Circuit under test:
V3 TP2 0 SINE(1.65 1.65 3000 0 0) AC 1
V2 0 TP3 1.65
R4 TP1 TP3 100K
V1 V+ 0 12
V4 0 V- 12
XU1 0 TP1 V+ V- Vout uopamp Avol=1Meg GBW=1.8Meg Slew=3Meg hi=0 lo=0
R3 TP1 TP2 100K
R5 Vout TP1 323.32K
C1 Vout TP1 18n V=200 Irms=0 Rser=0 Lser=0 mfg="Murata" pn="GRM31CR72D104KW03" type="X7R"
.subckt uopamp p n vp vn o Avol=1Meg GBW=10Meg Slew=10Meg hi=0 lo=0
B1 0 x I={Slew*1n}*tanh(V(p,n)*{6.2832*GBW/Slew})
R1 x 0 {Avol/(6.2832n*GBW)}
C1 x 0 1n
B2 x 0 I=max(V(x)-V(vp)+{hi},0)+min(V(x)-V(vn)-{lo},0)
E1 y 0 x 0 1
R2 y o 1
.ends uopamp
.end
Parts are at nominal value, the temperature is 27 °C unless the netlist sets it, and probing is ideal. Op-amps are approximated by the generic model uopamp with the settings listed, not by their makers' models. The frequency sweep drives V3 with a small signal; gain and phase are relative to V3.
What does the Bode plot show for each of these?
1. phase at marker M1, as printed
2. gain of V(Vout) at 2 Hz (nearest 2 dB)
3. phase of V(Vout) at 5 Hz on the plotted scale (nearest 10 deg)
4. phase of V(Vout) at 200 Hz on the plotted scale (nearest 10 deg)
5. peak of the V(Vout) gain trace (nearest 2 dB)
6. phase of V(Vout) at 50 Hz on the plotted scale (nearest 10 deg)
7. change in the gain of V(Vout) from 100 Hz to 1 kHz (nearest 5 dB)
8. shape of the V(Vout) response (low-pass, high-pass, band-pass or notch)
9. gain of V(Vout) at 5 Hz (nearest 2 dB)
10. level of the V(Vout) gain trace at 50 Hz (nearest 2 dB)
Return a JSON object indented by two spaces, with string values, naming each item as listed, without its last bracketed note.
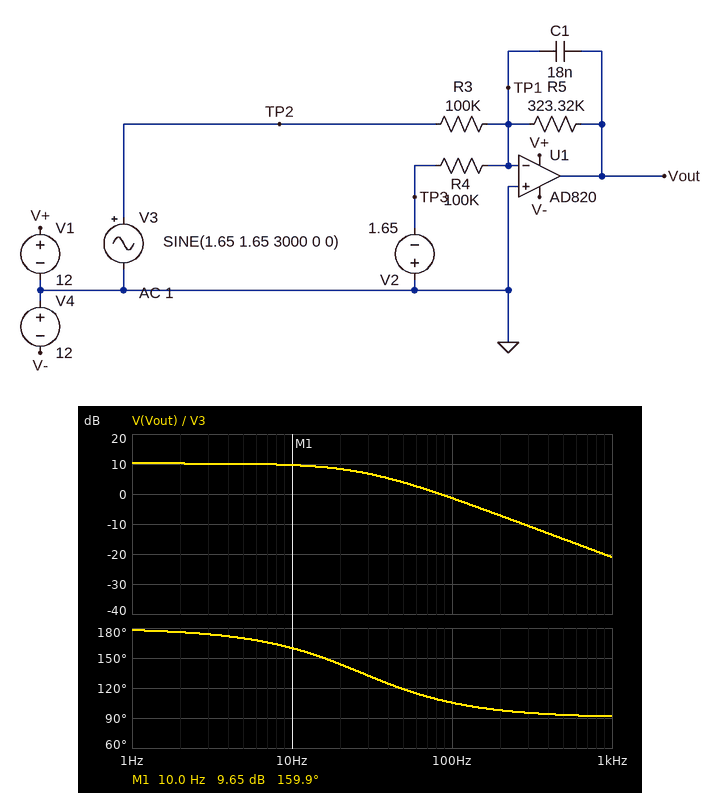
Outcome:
{
  "phase at marker M1, as printed": "159.9 deg",
  "gain of V(Vout) at 2 Hz": "10 dB",
  "phase of V(Vout) at 5 Hz on the plotted scale": "170 deg",
  "phase of V(Vout) at 200 Hz on the plotted scale": "100 deg",
  "peak of the V(Vout) gain trace": "10 dB",
  "phase of V(Vout) at 50 Hz on the plotted scale": "120 deg",
  "change in the gain of V(Vout) from 100 Hz to 1 kHz": "-20 dB",
  "shape of the V(Vout) response": "low-pass",
  "gain of V(Vout) at 5 Hz": "10 dB",
  "level of the V(Vout) gain trace at 50 Hz": "4 dB"
}
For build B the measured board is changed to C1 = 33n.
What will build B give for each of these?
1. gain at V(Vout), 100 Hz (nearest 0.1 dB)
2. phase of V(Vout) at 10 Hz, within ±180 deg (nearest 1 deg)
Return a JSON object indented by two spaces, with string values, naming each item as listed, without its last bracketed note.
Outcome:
{
  "gain at V(Vout), 100 Hz": "-6.4 dB",
  "phase of V(Vout) at 10 Hz, within ±180 deg": "146 deg"
}
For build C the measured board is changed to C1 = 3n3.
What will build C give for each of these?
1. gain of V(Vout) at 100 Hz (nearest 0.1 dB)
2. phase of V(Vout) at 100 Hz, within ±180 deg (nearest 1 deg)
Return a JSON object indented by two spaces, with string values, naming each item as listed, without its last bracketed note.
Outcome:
{
  "gain of V(Vout) at 100 Hz": "8.6 dB",
  "phase of V(Vout) at 100 Hz, within ±180 deg": "146 deg"
}
